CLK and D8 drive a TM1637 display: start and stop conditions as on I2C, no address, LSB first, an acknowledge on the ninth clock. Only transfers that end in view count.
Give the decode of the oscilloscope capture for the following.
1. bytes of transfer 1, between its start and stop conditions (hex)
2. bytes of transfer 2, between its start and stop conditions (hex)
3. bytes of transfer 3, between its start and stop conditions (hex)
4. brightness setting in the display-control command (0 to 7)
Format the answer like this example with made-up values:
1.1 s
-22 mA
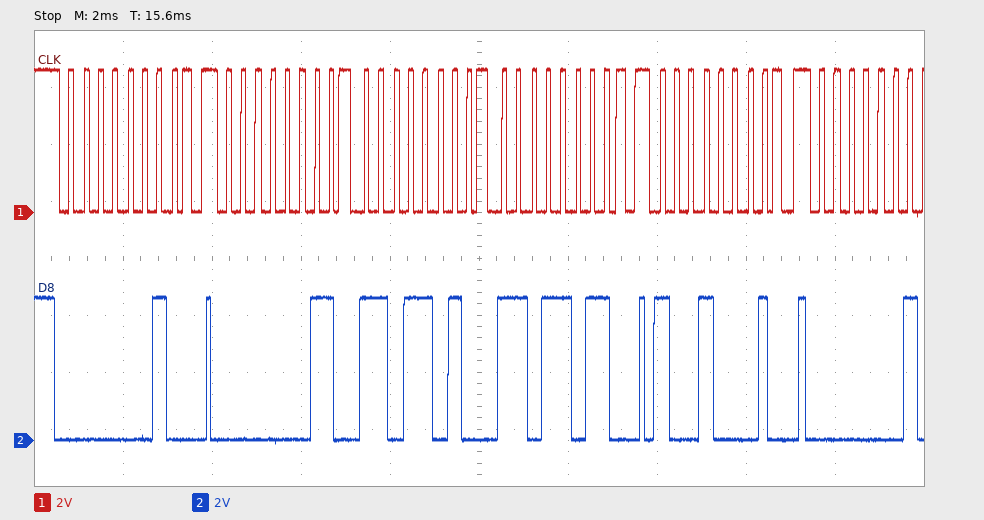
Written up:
40
C0 5B DB
89
1
